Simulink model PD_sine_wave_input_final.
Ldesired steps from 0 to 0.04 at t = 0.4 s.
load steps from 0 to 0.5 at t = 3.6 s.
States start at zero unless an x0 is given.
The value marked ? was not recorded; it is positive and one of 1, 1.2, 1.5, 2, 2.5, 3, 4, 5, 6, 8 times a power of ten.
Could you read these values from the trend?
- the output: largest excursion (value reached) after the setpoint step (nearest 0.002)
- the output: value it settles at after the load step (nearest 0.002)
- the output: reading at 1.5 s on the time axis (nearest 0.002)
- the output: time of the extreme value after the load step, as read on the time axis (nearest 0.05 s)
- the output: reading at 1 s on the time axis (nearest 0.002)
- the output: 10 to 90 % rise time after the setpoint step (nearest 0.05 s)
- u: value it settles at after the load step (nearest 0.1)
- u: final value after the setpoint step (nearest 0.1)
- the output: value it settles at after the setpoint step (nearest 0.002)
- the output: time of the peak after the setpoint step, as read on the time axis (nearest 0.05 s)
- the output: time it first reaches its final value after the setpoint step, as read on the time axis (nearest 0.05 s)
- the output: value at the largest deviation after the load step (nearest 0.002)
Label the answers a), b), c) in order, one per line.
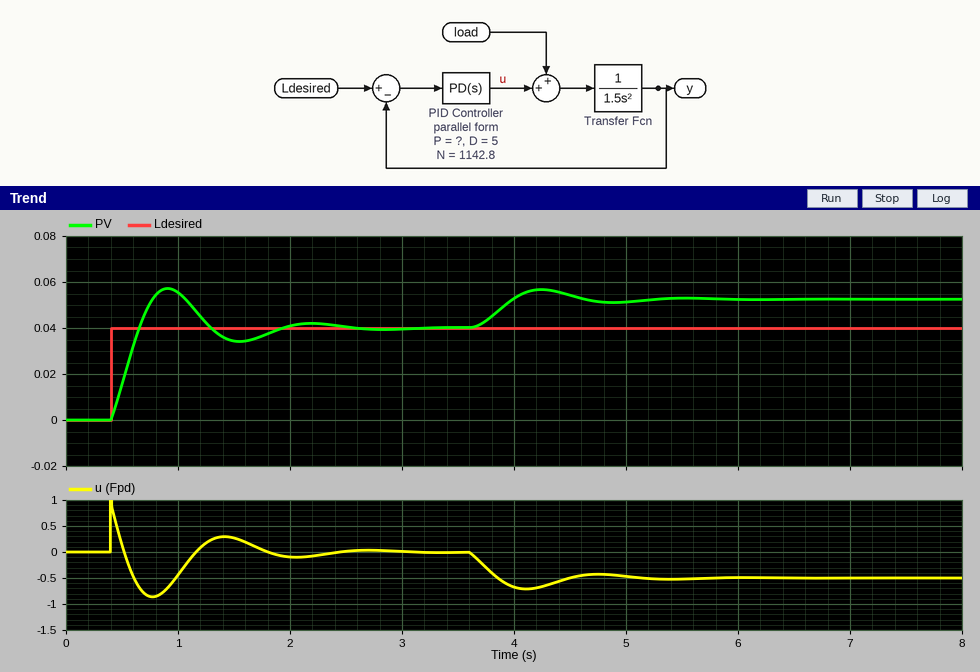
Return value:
a) 0.058
b) 0.052
c) 0.034
d) 4.25 s
e) 0.056
f) 0.20 s
g) -0.5
h) 0.0
i) 0.040
j) 0.90 s
k) 0.65 s
l) 0.056
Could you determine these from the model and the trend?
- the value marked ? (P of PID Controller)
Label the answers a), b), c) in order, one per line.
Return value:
a) 40
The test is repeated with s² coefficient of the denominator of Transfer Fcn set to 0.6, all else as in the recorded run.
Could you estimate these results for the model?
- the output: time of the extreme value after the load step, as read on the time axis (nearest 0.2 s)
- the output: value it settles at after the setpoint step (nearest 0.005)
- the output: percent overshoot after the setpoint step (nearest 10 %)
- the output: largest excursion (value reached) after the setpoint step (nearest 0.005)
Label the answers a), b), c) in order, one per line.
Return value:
a) 4.0 s
b) 0.040
c) 30 %
d) 0.050
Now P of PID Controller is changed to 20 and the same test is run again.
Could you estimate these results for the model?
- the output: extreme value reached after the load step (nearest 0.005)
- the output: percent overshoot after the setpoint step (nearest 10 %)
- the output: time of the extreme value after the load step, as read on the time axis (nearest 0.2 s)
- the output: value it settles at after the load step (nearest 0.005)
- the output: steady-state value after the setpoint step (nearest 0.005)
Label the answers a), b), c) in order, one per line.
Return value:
a) 0.070
b) 30 %
c) 4.6 s
d) 0.065
e) 0.040
